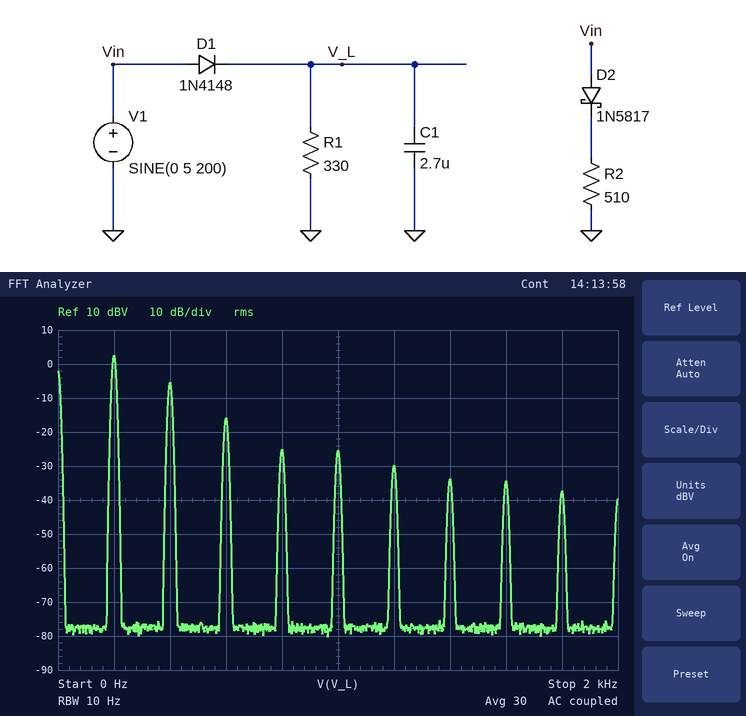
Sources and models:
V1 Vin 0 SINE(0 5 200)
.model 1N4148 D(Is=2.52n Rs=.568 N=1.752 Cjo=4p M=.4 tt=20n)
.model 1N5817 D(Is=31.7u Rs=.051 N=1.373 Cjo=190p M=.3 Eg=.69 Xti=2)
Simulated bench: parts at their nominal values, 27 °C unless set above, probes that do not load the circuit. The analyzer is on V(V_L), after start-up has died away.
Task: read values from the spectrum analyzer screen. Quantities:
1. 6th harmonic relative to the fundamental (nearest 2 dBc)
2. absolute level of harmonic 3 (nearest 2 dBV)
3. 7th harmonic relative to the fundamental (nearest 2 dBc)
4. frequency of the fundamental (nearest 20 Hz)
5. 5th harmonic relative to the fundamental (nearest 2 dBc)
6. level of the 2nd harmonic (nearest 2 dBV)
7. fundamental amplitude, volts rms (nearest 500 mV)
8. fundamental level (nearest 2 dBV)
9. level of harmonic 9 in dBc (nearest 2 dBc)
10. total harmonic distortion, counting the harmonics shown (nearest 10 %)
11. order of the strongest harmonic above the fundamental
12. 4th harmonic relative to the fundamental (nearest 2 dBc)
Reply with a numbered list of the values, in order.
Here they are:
1. -32 dBc
2. -16 dBV
3. -36 dBc
4. 200 Hz
5. -28 dBc
6. -6 dBV
7. 1.5 V
8. 2 dBV
9. -40 dBc
10. 40 %
11. 2
12. -28 dBc
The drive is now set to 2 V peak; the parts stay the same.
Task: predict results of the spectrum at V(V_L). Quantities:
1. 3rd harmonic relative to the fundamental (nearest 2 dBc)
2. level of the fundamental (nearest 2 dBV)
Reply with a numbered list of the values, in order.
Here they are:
1. -16 dBc
2. -8 dBV
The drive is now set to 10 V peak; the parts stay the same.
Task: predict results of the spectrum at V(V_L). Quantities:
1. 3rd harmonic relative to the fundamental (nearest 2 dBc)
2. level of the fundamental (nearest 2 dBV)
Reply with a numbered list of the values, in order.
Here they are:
1. -20 dBc
2. 10 dBV
